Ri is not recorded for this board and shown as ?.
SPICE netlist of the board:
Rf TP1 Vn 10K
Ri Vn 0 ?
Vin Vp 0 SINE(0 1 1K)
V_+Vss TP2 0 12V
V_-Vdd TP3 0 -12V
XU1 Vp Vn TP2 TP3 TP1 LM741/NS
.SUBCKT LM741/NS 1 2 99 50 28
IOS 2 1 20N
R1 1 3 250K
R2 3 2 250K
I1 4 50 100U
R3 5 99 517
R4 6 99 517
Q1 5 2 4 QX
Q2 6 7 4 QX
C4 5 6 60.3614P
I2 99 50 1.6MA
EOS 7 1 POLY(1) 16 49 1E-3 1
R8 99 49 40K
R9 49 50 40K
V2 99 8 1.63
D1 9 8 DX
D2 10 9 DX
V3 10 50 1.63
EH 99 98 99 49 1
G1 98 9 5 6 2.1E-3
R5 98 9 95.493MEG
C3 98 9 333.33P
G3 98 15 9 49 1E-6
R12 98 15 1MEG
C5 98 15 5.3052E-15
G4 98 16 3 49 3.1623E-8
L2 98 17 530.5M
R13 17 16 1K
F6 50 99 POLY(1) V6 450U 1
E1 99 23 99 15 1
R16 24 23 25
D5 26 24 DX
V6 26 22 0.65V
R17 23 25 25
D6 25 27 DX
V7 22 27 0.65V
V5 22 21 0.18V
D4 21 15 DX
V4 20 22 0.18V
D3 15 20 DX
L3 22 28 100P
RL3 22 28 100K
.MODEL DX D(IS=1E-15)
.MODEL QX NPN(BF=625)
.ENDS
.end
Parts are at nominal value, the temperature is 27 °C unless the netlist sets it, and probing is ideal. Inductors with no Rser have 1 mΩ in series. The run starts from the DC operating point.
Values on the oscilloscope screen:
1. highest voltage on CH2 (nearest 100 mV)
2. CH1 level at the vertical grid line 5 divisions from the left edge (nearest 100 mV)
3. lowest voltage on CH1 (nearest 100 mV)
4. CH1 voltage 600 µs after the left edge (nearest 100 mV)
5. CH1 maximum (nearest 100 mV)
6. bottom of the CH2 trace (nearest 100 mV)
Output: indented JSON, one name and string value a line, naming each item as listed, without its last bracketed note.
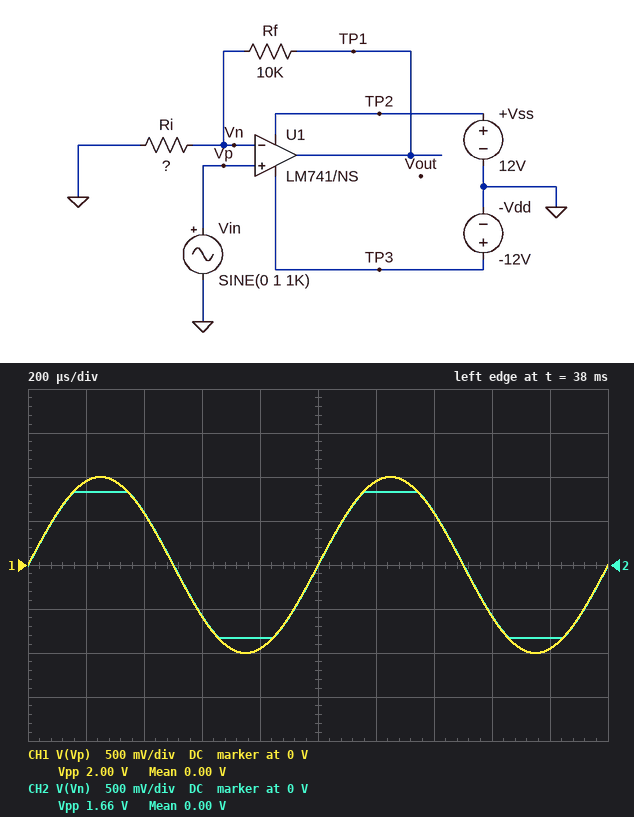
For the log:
{
  "highest voltage on CH2": "800 mV",
  "CH1 level at the vertical grid line 5 divisions from the left edge": "0 V",
  "lowest voltage on CH1": "-1.0 V",
  "CH1 voltage 600 µs after the left edge": "-600 mV",
  "CH1 maximum": "1.0 V",
  "bottom of the CH2 trace": "-800 mV"
}
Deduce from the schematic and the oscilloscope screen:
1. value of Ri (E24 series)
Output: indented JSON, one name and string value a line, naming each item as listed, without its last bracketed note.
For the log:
{
  "value of Ri": "820 Ω"
}
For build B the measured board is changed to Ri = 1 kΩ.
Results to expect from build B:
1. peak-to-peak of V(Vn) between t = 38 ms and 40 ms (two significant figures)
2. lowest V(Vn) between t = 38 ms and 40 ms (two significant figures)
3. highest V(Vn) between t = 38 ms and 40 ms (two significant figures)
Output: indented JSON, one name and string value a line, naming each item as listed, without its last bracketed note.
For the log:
{
  "peak-to-peak of V(Vn) between t = 38 ms and 40 ms": "2.0 V",
  "lowest V(Vn) between t = 38 ms and 40 ms": "-990 mV",
  "highest V(Vn) between t = 38 ms and 40 ms": "990 mV"
}
